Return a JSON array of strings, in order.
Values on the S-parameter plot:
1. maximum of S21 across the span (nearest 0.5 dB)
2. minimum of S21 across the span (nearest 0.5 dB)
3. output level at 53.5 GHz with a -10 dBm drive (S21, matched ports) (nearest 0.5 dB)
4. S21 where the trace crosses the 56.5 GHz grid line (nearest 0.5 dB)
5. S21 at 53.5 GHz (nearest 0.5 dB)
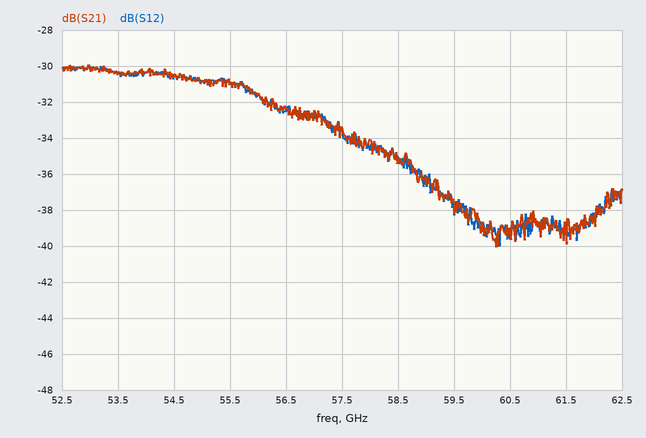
["-30.0 dB", "-40.0 dB", "-40.5 dBm", "-32.5 dB", "-30.5 dB"]
